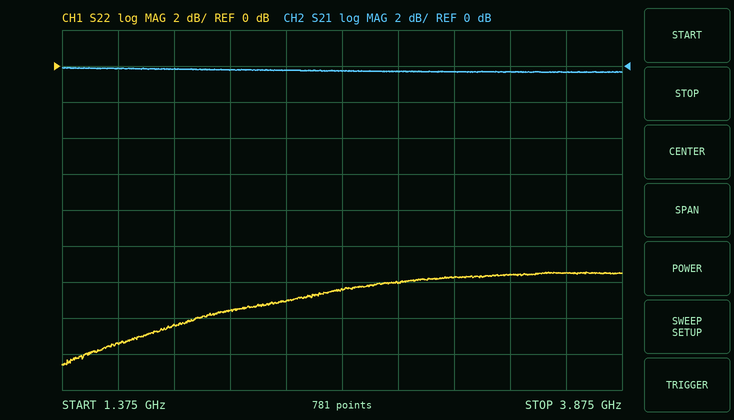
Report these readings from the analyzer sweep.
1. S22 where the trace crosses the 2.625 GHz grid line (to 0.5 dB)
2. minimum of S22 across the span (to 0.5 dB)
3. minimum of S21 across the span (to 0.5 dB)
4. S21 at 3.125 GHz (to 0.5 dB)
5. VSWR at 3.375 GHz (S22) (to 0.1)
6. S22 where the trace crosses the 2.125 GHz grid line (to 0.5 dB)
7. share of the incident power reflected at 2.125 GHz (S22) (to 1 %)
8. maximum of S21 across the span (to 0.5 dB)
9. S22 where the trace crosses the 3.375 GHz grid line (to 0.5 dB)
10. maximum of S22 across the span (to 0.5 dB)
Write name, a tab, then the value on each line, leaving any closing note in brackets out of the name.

S22 where the trace crosses the 2.625 GHz grid line	-12.5 dB
minimum of S22 across the span	-16.5 dB
minimum of S21 across the span	-0.5 dB
S21 at 3.125 GHz	-0.5 dB
VSWR at 3.375 GHz (S22)	1.7
S22 where the trace crosses the 2.125 GHz grid line	-13.5 dB
share of the incident power reflected at 2.125 GHz (S22)	4 %
maximum of S21 across the span	0.0 dB
S22 where the trace crosses the 3.375 GHz grid line	-11.5 dB
maximum of S22 across the span	-11.5 dB
